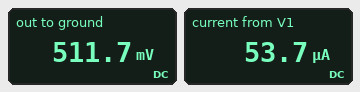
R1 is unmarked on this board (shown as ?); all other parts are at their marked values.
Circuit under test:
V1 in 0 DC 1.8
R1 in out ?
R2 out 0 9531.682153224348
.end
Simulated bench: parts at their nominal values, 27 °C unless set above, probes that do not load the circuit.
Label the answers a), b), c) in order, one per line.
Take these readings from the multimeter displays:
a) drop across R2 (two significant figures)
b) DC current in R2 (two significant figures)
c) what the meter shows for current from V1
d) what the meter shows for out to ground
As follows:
a) 510 mV
b) 54 µA
c) 53.7 µA
d) 511.7 mV
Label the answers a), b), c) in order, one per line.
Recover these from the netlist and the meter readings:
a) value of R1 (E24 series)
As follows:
a) 24 kΩ
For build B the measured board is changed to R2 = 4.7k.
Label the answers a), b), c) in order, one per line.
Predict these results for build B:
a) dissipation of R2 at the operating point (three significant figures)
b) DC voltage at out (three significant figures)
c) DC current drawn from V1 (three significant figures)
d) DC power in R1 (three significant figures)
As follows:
a) 18.5 µW
b) 295 mV
c) 62.7 µA
d) 94.4 µW
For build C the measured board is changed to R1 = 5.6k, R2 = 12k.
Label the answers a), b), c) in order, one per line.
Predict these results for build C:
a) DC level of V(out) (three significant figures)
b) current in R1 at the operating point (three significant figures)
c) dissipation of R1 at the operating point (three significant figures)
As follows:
a) 1.23 V
b) 102 µA
c) 58.6 µW
